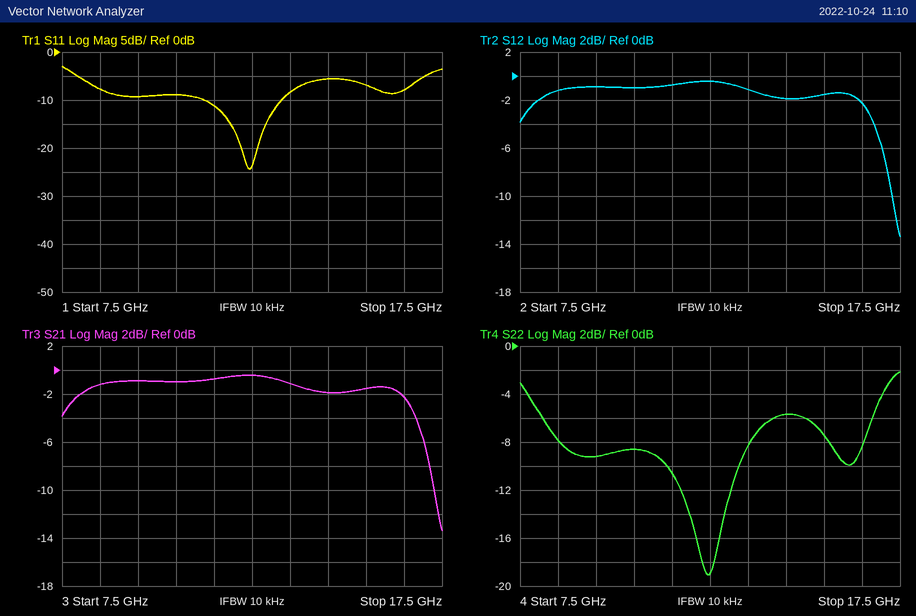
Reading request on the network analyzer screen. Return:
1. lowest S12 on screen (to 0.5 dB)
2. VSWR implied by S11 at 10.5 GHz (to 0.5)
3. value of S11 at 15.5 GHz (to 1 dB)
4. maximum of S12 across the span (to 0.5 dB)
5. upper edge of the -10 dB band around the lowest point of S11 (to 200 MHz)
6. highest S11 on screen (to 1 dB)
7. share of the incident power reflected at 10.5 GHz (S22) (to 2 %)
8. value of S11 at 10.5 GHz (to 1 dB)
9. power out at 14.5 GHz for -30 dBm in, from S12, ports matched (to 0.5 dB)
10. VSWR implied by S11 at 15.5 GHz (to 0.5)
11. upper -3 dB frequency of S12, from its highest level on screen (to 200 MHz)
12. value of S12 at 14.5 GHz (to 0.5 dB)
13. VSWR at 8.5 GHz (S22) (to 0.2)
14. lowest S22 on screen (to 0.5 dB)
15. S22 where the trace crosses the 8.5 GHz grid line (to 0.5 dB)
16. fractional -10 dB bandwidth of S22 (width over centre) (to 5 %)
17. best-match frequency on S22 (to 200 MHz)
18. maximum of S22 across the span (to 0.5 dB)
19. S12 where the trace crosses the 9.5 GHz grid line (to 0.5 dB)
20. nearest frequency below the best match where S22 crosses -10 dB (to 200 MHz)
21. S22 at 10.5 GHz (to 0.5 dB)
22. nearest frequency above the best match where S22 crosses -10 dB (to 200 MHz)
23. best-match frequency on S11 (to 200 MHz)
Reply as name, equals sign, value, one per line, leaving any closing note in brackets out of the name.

lowest S12 on screen = -13.5 dB
VSWR implied by S11 at 10.5 GHz = 2.0
value of S11 at 15.5 GHz = -7 dB
maximum of S12 across the span = -0.5 dB
upper edge of the -10 dB band around the lowest point of S11 = 13.2 GHz
highest S11 on screen = -3 dB
share of the incident power reflected at 10.5 GHz (S22) = 14 %
value of S11 at 10.5 GHz = -9 dB
power out at 14.5 GHz for -30 dBm in, from S12, ports matched = -32.0 dBm
VSWR implied by S11 at 15.5 GHz = 2.5
upper -3 dB frequency of S12, from its highest level on screen = 16.8 GHz
value of S12 at 14.5 GHz = -2.0 dB
VSWR at 8.5 GHz (S22) = 2.4
lowest S22 on screen = -19.0 dB
S22 where the trace crosses the 8.5 GHz grid line = -8.0 dB
fractional -10 dB bandwidth of S22 (width over centre) = 15 %
best-match frequency on S22 = 12.4 GHz
maximum of S22 across the span = -2.0 dB
S12 where the trace crosses the 9.5 GHz grid line = -1.0 dB
nearest frequency below the best match where S22 crosses -10 dB = 11.4 GHz
S22 at 10.5 GHz = -8.5 dB
nearest frequency above the best match where S22 crosses -10 dB = 13.2 GHz
best-match frequency on S11 = 12.4 GHz
